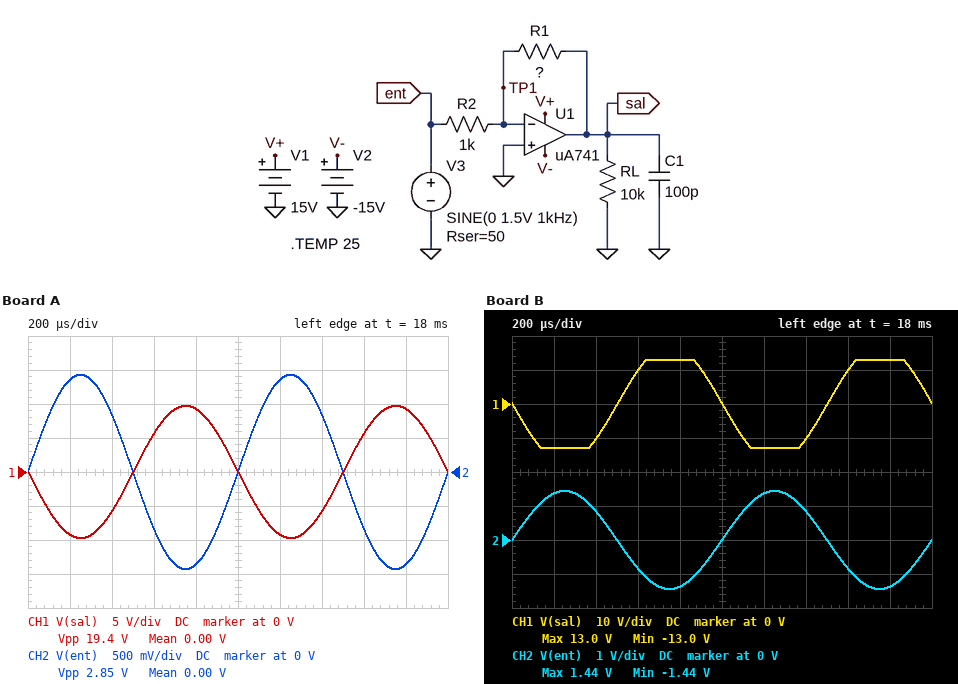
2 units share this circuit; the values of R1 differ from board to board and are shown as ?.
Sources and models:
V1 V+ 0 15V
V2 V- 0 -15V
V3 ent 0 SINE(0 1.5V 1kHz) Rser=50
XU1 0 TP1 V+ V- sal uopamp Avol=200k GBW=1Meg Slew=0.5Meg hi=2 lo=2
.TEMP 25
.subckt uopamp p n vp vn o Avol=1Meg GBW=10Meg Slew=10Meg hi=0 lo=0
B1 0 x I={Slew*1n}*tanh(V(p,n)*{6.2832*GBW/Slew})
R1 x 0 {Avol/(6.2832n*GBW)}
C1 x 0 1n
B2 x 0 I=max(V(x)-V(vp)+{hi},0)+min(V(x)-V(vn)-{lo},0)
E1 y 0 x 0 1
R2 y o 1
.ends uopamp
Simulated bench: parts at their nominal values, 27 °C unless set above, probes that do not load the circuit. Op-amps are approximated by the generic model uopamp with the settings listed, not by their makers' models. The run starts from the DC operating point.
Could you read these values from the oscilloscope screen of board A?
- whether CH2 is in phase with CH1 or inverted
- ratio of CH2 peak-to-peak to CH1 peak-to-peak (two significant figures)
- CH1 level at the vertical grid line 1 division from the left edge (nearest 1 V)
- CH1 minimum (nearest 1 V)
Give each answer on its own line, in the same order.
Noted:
inverted
0.15
-9 V
-10 V
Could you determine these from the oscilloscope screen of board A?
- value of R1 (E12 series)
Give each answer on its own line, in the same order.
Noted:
6.8 kΩ
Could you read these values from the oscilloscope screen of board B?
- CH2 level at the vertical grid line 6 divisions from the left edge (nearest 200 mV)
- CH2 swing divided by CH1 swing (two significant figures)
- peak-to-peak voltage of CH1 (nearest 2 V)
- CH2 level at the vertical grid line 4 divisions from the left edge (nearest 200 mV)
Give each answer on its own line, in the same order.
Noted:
1.4 V
0.11
26 V
-1.4 V
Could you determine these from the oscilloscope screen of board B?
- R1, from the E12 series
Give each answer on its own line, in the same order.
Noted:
12 kΩ
